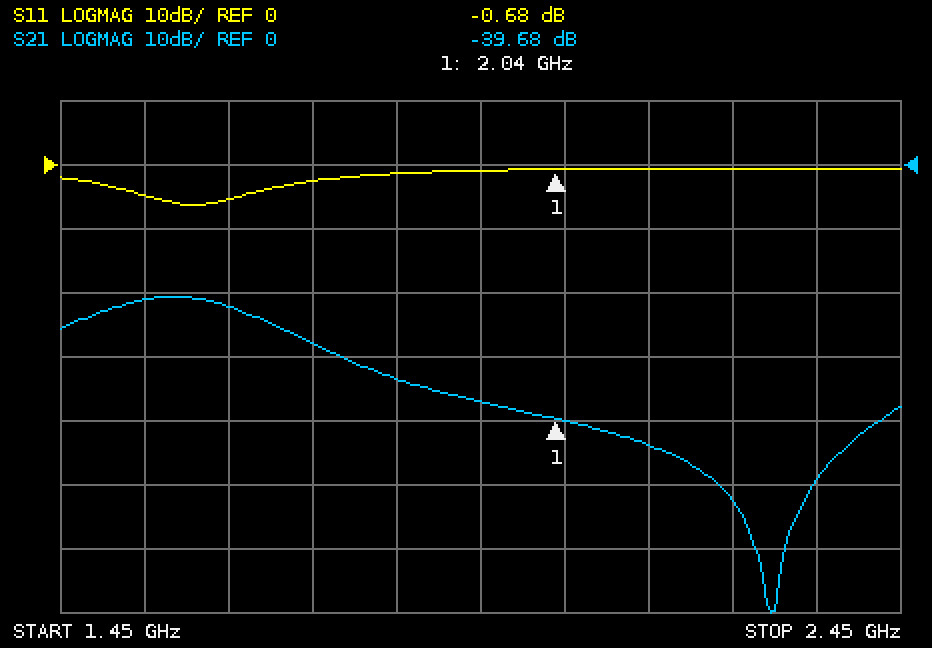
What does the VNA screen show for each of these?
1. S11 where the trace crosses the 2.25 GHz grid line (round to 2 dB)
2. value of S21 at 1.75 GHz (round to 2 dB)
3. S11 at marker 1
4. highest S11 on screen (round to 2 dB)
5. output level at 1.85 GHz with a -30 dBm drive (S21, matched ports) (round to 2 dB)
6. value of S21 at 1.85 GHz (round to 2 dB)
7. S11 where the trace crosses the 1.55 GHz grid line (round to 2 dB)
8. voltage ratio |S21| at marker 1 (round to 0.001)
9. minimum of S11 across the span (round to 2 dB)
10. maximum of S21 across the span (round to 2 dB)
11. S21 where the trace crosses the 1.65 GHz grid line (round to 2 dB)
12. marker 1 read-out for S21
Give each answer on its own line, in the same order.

0 dB
-28 dB
-0.68 dB
0 dB
-64 dBm
-34 dB
-4 dB
0.010
-6 dB
-20 dB
-22 dB
-39.68 dB
